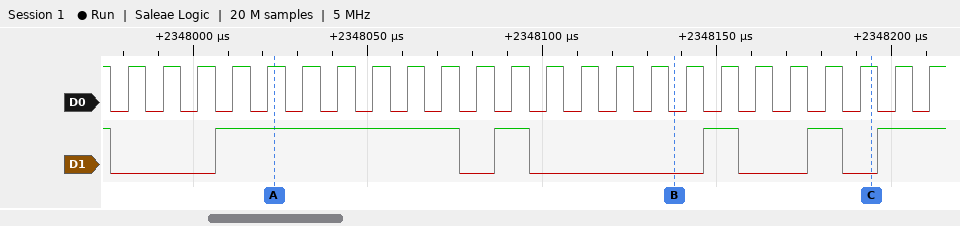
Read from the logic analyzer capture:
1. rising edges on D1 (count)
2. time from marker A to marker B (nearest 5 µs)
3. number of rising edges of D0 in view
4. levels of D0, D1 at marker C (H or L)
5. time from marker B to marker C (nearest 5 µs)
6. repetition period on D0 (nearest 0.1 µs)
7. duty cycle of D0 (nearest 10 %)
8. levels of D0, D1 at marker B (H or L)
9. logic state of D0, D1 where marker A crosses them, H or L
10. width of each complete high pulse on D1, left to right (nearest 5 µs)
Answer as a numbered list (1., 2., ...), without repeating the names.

1. 5
2. 115 µs
3. 24
4. D0=H, D1=L
5. 55 µs
6. 10 µs
7. 50 %
8. D0=L, D1=L
9. D0=H, D1=H
10. 70 µs, 10 µs, 10 µs, 10 µs
